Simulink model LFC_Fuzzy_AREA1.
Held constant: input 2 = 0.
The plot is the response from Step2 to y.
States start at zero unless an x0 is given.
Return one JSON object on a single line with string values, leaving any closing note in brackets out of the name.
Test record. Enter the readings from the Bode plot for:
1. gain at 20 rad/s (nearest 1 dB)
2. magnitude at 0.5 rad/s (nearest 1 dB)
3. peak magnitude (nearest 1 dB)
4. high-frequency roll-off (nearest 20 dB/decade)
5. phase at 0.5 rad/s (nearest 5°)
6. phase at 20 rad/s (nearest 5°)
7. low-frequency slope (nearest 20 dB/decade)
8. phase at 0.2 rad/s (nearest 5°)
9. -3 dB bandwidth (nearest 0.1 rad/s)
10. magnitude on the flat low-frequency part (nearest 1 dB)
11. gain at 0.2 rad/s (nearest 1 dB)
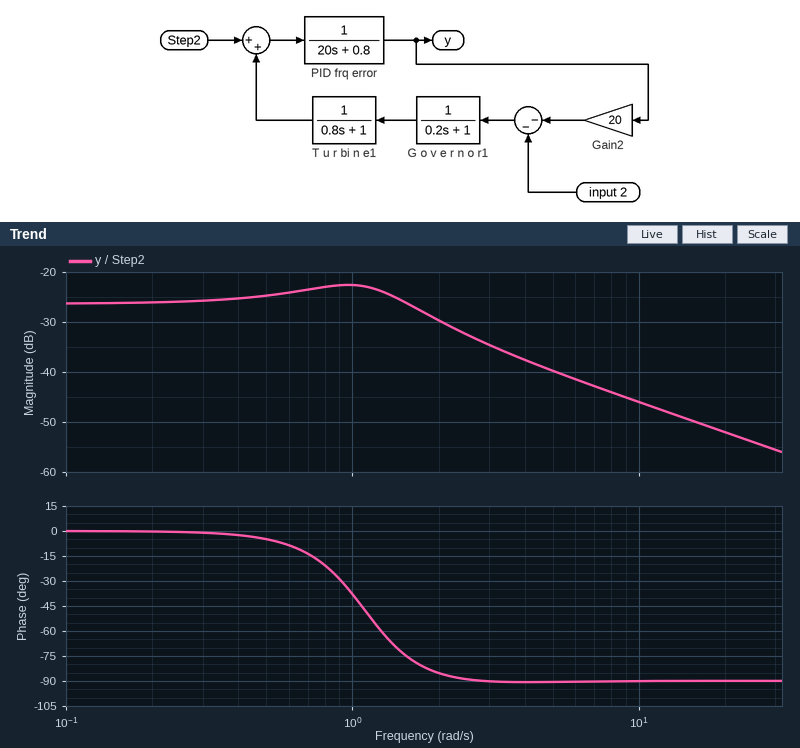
{"gain at 20 rad/s": "-52 dB", "magnitude at 0.5 rad/s": "-25 dB", "peak magnitude": "-23 dB", "high-frequency roll-off": "-20 dB/decade", "phase at 0.5 rad/s": "-5°", "phase at 20 rad/s": "-90°", "low-frequency slope": "0 dB/decade", "phase at 0.2 rad/s": "0°", "-3 dB bandwidth": "1.9 rad/s", "magnitude on the flat low-frequency part": "-26 dB", "gain at 0.2 rad/s": "-26 dB"}
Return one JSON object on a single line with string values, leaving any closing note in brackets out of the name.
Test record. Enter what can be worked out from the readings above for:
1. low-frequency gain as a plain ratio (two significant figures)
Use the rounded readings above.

{"low-frequency gain as a plain ratio": "0.050"}
